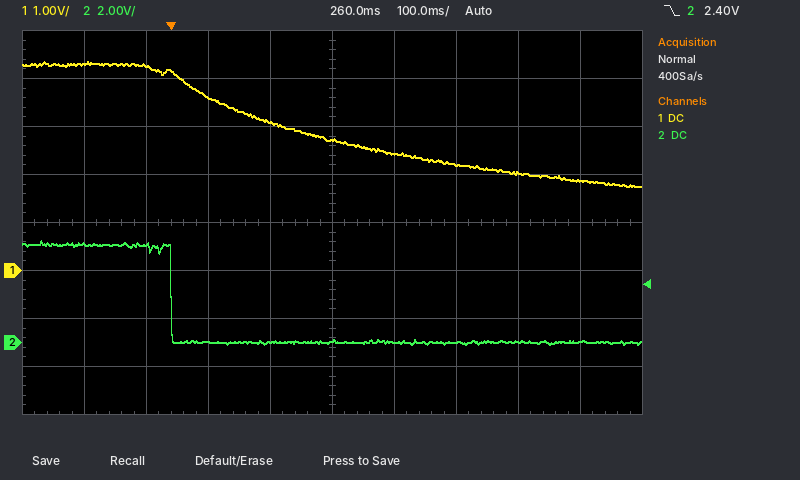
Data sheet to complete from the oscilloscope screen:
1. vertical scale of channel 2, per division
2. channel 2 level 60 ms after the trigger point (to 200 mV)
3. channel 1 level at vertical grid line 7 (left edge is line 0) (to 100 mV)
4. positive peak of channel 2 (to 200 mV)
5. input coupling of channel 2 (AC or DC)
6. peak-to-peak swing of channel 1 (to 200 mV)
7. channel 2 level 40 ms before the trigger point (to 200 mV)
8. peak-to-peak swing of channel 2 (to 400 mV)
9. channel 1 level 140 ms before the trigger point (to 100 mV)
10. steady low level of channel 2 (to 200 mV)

2 V
0.0 V
2.2 V
4.2 V
DC
2.6 V
4.0 V
4.4 V
4.3 V
0.0 V
